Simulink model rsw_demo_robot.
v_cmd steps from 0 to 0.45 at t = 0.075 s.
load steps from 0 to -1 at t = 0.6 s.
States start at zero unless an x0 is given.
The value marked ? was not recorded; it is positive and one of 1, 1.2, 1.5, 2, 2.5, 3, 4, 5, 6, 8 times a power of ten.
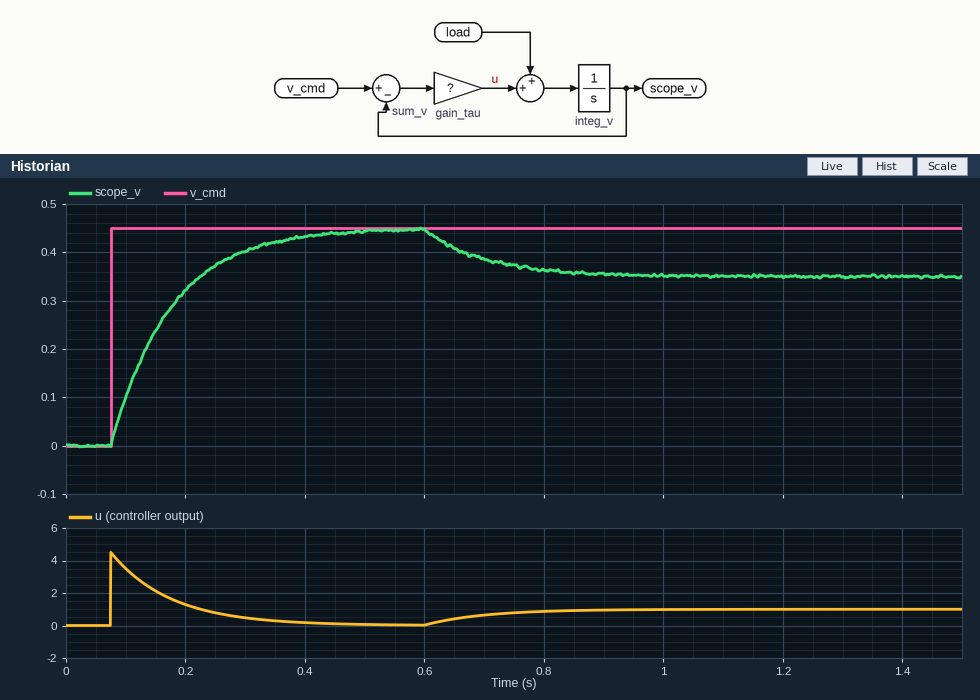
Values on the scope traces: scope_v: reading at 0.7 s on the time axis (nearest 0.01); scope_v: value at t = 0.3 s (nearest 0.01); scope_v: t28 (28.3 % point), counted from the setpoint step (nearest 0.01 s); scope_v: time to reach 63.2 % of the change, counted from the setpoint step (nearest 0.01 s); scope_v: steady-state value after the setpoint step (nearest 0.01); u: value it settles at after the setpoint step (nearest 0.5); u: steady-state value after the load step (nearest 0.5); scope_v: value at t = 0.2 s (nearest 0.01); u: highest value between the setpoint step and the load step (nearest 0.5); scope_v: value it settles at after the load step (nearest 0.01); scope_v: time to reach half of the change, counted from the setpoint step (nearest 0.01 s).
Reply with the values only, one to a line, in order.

0.39
0.40
0.03 s
0.10 s
0.45
0.0
1.0
0.32
4.5
0.35
0.07 s
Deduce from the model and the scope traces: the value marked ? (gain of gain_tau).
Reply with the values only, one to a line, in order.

10
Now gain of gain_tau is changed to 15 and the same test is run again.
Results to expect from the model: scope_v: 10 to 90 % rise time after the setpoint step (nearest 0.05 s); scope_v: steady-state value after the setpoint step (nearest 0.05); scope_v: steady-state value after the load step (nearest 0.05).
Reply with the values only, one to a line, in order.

0.15 s
0.45
0.40
